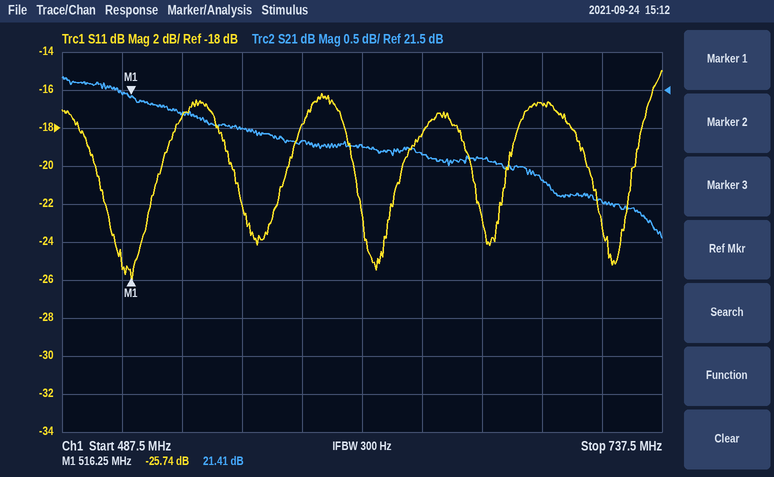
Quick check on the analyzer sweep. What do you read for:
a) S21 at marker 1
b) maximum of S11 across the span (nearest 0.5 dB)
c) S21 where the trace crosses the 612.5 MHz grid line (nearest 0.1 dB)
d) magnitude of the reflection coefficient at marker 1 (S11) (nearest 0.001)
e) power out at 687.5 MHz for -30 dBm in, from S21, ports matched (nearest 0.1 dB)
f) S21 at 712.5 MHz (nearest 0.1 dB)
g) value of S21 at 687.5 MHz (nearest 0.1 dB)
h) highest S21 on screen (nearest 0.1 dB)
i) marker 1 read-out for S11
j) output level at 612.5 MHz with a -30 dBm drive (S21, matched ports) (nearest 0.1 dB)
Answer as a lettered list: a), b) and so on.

a) 21.41 dB
b) -15.0 dB
c) 20.8 dB
d) 0.052
e) -9.7 dBm
f) 20.0 dB
g) 20.3 dB
h) 21.7 dB
i) -25.74 dB
j) -9.2 dBm
